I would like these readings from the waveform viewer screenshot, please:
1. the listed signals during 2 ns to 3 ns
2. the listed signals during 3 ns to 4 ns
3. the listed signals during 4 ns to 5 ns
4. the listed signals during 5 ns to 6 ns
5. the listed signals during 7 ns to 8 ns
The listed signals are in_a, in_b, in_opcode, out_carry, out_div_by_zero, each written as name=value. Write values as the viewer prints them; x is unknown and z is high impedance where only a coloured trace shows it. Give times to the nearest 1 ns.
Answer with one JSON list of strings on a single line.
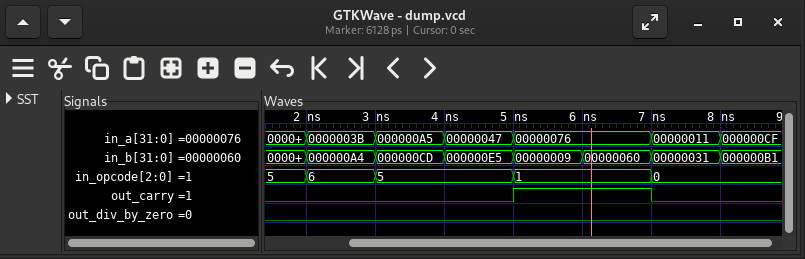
["in_a=0000003B, in_b=000000A4, in_opcode=6, out_carry=0, out_div_by_zero=0", "in_a=000000A5, in_b=000000CD, in_opcode=5, out_carry=0, out_div_by_zero=0", "in_a=00000047, in_b=000000E5, in_opcode=5, out_carry=0, out_div_by_zero=0", "in_a=00000076, in_b=00000009, in_opcode=1, out_carry=1, out_div_by_zero=0", "in_a=00000011, in_b=00000031, in_opcode=0, out_carry=0, out_div_by_zero=0"]
